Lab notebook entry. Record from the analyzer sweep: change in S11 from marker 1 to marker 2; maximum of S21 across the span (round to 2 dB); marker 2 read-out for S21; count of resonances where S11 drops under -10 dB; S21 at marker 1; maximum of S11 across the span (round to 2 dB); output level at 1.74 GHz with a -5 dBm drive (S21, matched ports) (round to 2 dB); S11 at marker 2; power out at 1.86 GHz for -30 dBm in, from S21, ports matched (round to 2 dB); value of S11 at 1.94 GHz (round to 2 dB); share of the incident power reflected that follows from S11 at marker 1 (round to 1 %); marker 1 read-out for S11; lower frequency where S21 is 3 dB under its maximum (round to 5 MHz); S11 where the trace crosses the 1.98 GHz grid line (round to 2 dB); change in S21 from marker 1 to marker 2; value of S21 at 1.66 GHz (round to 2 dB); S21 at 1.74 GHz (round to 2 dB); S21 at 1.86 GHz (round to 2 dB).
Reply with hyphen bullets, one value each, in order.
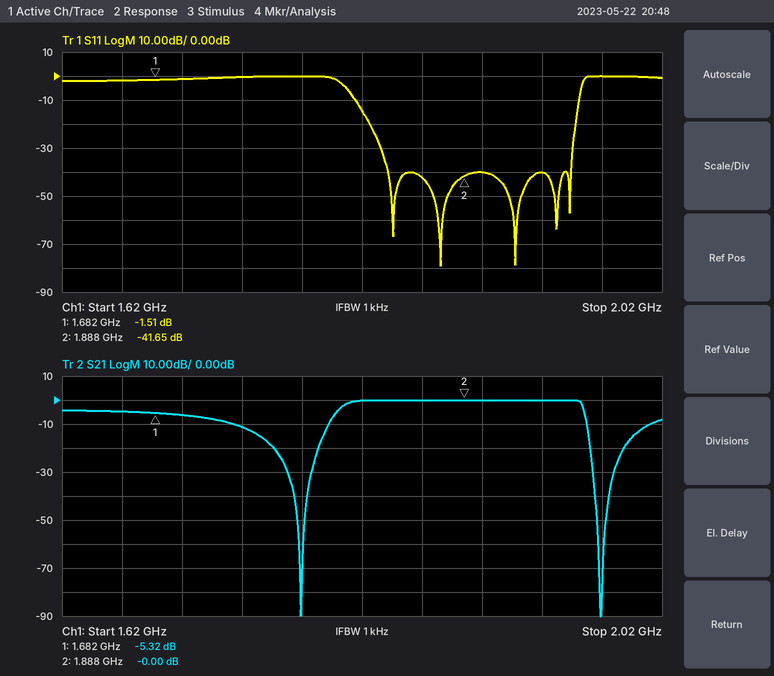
- -40.14 dB
- 0 dB
- -0.00 dB
- 5
- -5.32 dB
- 0 dB
- -16 dBm
- -41.65 dB
- -30 dBm
- -40 dB
- 71 %
- -1.51 dB
- 1.805 GHz
- 0 dB
- 5.32 dB
- -4 dB
- -12 dB
- 0 dB
